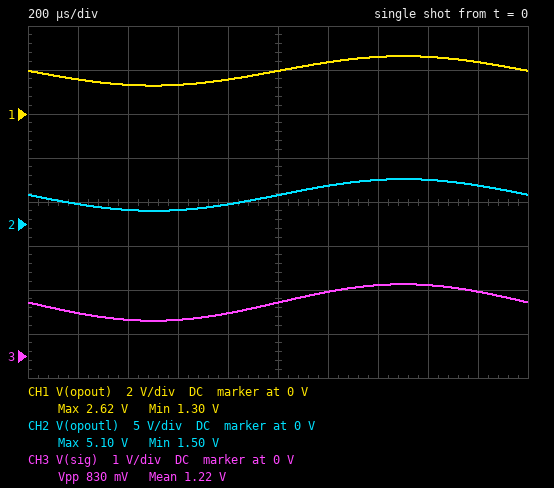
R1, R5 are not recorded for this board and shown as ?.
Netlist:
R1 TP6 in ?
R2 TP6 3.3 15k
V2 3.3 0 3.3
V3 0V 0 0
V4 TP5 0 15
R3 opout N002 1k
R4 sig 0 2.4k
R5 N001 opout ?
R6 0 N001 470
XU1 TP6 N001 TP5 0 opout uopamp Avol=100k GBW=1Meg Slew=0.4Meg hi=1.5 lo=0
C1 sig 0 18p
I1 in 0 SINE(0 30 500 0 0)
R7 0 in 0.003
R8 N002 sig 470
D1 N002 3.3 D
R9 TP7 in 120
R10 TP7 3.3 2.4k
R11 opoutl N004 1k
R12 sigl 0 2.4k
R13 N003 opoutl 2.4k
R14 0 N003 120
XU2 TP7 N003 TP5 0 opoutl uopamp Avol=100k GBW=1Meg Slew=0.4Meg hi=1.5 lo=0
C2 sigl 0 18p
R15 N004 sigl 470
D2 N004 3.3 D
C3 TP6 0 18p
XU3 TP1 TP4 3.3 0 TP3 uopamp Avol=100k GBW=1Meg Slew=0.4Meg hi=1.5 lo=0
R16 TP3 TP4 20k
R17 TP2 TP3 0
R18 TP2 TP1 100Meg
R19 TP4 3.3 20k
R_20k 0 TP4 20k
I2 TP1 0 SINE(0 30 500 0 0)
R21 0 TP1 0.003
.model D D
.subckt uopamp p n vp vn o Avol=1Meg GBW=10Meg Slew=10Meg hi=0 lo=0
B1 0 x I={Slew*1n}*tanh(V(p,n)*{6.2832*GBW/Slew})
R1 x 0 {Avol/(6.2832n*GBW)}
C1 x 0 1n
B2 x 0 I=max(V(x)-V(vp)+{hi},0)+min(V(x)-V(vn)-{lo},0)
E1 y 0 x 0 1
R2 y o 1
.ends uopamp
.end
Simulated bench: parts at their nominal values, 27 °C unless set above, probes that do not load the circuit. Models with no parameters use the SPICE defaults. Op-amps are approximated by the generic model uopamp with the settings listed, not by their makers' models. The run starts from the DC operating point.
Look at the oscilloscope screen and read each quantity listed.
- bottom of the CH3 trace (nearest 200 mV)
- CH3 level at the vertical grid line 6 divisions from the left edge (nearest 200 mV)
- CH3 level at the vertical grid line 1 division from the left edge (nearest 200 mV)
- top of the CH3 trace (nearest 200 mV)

800 mV
1.4 V
1.0 V
1.6 V
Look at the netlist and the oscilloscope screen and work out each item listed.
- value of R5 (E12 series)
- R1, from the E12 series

3.3 kΩ
1.2 kΩ
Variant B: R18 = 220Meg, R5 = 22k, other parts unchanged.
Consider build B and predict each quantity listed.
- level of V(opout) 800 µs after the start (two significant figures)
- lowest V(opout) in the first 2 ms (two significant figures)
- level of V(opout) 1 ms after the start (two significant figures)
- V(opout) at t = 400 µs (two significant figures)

9.3 V
7.7 V
12 V
7.9 V
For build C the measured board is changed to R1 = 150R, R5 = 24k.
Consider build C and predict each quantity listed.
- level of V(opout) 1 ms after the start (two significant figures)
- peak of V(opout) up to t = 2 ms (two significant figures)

1.6 V
6.3 V
